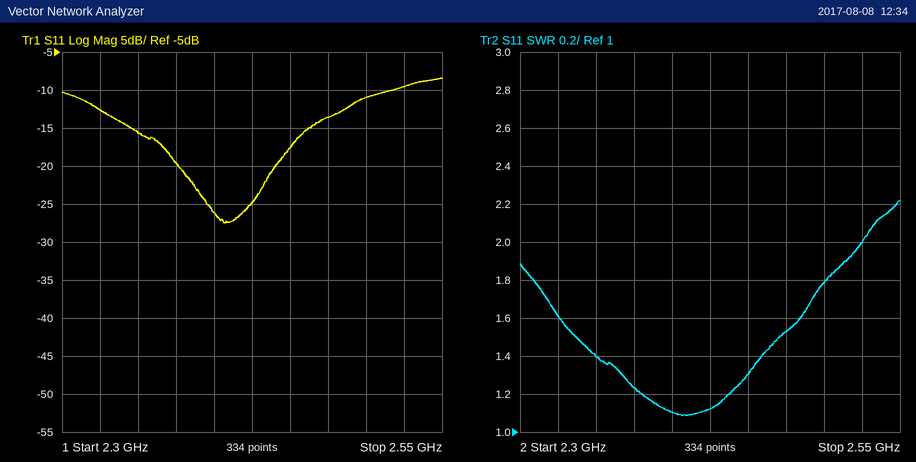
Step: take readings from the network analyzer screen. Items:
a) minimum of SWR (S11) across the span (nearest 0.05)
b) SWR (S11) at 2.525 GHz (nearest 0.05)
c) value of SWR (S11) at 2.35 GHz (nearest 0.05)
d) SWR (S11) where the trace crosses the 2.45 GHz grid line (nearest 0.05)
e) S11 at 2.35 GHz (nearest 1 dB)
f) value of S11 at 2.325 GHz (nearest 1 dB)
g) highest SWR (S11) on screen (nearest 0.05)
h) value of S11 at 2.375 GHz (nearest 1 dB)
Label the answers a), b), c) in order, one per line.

a) 1.10
b) 2.00
c) 1.40
d) 1.30
e) -16 dB
f) -13 dB
g) 2.20
h) -20 dB
